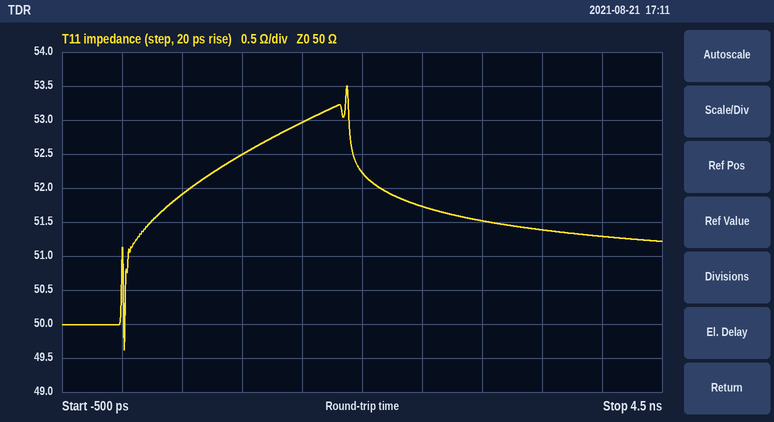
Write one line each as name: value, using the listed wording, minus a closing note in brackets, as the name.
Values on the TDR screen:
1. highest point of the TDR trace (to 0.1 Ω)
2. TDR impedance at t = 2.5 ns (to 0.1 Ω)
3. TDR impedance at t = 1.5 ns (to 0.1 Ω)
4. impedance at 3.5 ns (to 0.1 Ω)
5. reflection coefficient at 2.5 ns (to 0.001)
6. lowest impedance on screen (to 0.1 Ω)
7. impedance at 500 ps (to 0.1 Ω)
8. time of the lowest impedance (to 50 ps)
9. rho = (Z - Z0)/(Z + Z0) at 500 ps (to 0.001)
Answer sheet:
highest point of the TDR trace: 53.5 Ω
TDR impedance at t = 2.5 ns: 51.7 Ω
TDR impedance at t = 1.5 ns: 53.0 Ω
impedance at 3.5 ns: 51.4 Ω
reflection coefficient at 2.5 ns: +0.017
lowest impedance on screen: 49.6 Ω
impedance at 500 ps: 51.9 Ω
time of the lowest impedance: 0 ps
rho = (Z - Z0)/(Z + Z0) at 500 ps: +0.019
